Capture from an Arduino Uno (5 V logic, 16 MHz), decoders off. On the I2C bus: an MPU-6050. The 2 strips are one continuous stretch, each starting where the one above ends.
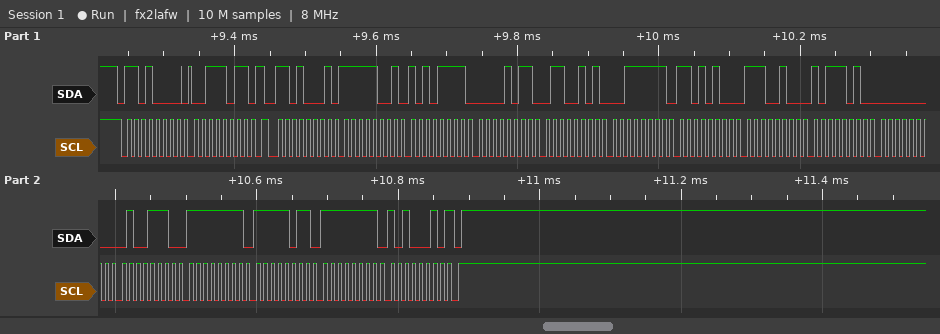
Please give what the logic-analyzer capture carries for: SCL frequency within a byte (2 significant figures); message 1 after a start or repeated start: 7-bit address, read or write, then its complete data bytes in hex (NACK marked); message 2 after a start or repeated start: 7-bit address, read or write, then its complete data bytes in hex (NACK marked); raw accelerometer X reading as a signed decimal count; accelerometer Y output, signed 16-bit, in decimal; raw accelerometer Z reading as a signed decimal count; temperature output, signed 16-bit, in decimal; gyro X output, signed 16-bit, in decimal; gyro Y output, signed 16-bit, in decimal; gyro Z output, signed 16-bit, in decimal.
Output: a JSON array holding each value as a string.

["100 kHz", "0x68 write: 3B", "0x68 read: F9 AF 0B 65 3F D4 E4 BA 00 4E FF FB FF A2 NACK", "-1617", "2917", "16340", "-6982", "78", "-5", "-94"]
